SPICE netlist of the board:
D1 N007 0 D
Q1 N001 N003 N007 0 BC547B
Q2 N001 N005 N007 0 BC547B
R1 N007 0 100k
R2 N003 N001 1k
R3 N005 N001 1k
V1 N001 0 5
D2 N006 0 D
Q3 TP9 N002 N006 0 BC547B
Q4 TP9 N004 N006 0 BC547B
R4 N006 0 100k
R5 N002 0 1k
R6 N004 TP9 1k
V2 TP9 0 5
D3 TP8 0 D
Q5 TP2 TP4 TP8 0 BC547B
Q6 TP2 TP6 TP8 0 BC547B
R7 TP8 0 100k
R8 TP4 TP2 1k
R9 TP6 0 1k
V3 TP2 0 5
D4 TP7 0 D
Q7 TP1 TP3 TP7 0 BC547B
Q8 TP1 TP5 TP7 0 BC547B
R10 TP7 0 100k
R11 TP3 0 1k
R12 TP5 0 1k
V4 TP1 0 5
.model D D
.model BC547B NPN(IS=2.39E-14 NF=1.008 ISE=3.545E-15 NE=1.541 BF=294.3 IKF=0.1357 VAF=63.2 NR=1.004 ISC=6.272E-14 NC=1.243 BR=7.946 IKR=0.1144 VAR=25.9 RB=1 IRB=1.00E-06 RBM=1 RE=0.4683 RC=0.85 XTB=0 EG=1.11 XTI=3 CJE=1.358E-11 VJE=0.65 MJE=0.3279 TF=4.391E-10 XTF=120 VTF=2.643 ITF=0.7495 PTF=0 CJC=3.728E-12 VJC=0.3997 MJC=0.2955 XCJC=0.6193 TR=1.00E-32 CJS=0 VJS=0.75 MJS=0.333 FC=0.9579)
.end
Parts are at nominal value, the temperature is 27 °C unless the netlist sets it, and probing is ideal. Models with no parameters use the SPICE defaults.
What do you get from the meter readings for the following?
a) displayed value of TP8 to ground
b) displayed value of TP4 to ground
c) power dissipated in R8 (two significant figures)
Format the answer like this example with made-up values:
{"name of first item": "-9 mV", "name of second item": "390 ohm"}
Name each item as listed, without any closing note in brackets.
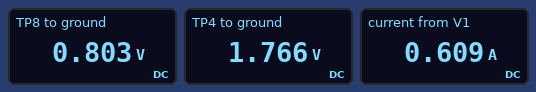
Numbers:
{"displayed value of TP8 to ground": "0.803 V", "displayed value of TP4 to ground": "1.766 V", "power dissipated in R8": "10 mW"}
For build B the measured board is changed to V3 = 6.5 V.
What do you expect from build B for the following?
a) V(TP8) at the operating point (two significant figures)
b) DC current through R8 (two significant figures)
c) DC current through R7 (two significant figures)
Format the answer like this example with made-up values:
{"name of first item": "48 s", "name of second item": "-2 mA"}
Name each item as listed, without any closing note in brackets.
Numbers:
{"V(TP8) at the operating point": "810 mV", "DC current through R8": "4.7 mA", "DC current through R7": "8.1 µA"}
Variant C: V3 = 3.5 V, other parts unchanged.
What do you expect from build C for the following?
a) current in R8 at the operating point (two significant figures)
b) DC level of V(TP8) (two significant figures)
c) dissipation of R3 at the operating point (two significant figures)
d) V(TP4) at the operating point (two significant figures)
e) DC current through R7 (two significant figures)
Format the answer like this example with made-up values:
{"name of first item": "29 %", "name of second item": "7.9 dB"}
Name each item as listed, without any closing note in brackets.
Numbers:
{"current in R8 at the operating point": "1.8 mA", "DC level of V(TP8)": "790 mV", "dissipation of R3 at the operating point": "10 mW", "V(TP4) at the operating point": "1.7 V", "DC current through R7": "7.9 µA"}
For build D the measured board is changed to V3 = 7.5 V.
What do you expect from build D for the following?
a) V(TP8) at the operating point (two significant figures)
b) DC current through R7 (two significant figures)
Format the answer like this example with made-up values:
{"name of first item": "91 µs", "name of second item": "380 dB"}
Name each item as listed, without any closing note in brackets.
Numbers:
{"V(TP8) at the operating point": "810 mV", "DC current through R7": "8.1 µA"}
